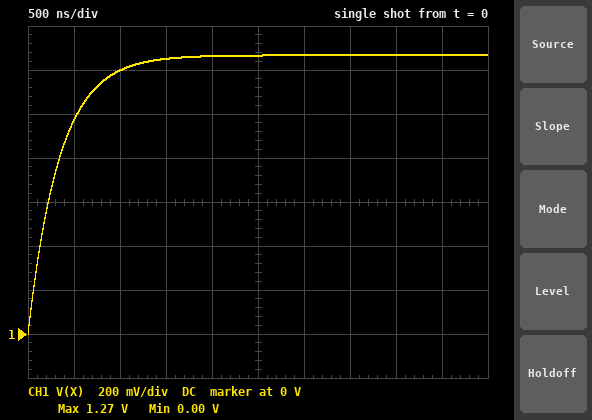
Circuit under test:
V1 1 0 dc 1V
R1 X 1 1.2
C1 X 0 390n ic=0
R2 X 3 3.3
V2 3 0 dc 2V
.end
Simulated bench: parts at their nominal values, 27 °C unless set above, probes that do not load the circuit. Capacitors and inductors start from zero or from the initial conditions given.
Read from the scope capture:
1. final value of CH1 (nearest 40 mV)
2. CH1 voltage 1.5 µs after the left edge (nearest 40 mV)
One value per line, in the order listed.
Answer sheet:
1.28 V
1.24 V
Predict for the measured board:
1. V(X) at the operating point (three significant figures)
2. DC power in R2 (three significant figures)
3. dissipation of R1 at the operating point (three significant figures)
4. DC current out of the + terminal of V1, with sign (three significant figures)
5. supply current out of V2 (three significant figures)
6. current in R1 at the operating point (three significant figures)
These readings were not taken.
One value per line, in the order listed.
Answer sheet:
1.27 V
163 mW
59.3 mW
-222 mA
222 mA
222 mA
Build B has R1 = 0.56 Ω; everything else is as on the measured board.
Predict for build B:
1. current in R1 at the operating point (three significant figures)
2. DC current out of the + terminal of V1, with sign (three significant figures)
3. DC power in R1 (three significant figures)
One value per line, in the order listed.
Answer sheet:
259 mA
-259 mA
37.6 mW
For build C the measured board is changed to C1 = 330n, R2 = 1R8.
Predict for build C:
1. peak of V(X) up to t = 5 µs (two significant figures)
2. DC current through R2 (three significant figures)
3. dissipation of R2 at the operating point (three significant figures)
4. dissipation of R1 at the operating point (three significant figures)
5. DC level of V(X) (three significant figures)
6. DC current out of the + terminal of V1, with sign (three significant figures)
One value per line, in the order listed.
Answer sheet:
1.4 V
333 mA
200 mW
133 mW
1.40 V
-333 mA
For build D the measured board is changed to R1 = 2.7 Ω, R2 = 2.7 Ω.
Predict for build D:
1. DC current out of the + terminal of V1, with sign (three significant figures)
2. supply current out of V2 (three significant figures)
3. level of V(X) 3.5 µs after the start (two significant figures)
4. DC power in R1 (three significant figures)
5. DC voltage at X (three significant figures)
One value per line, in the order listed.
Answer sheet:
-185 mA
185 mA
1.5 V
92.6 mW
1.50 V
